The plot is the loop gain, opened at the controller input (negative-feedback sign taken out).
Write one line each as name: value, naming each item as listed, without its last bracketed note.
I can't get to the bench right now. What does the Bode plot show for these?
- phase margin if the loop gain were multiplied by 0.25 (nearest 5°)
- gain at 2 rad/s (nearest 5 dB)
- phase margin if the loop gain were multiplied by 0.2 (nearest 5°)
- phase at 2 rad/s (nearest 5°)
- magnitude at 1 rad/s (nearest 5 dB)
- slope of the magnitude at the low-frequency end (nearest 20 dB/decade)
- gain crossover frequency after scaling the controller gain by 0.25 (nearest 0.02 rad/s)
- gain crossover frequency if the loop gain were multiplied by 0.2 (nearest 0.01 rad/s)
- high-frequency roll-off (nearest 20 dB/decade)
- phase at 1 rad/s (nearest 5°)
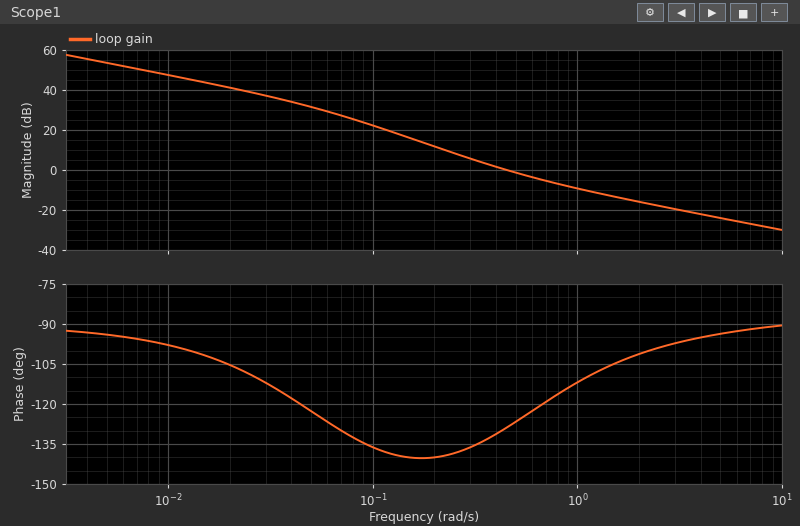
phase margin if the loop gain were multiplied by 0.25: 40°
gain at 2 rad/s: -15 dB
phase margin if the loop gain were multiplied by 0.2: 40°
phase at 2 rad/s: -100°
magnitude at 1 rad/s: -10 dB
slope of the magnitude at the low-frequency end: -20 dB/decade
gain crossover frequency after scaling the controller gain by 0.25: 0.20 rad/s
gain crossover frequency if the loop gain were multiplied by 0.2: 0.17 rad/s
high-frequency roll-off: -20 dB/decade
phase at 1 rad/s: -110°
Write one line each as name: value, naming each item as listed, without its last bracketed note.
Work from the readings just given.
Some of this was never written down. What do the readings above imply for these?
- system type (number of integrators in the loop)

system type: 1
